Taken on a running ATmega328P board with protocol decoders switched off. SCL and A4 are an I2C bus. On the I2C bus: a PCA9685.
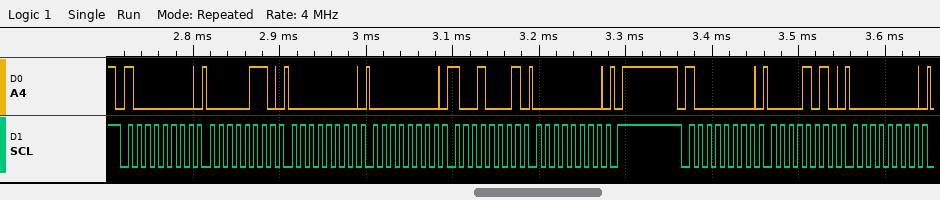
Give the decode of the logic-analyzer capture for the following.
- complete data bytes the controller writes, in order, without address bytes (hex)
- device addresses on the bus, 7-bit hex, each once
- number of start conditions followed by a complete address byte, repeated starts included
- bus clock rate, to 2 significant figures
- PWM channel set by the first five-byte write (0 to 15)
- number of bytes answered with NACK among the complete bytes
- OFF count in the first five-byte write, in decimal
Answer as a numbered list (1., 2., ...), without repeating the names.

1. 06 00 00 91 00 0A 00
2. 0x40
3. 2
4. 100 kHz
5. 0
6. 0
7. 145
